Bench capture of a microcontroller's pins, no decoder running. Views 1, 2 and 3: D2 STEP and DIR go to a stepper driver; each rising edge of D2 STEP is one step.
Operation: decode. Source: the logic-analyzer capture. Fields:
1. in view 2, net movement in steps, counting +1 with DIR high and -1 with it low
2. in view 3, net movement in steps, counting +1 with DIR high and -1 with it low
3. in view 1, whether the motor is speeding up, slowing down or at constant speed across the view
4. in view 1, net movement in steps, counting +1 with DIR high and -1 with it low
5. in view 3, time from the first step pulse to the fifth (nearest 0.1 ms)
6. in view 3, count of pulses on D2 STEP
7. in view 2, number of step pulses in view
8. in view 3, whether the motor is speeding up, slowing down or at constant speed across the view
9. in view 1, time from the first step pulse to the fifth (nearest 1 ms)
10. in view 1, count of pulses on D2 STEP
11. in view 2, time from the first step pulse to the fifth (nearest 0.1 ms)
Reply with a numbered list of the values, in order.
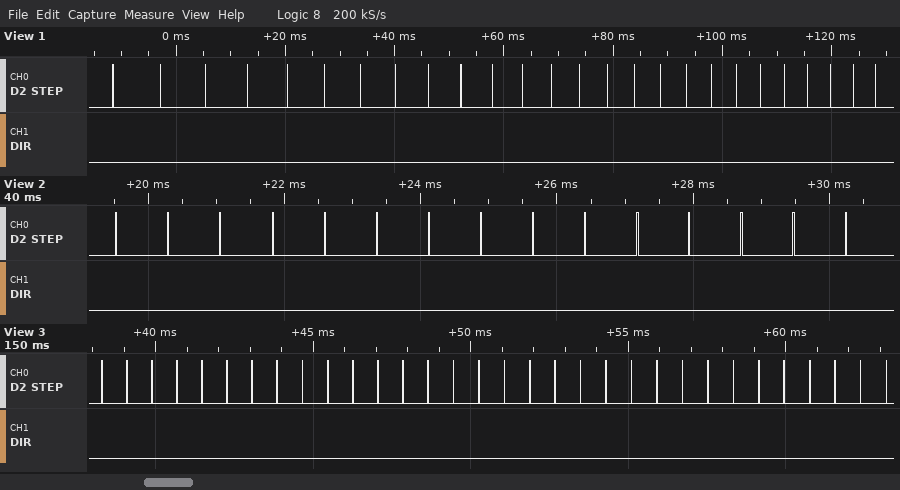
1. -15
2. -32
3. speeding up
4. -26
5. 3.2 ms
6. 32
7. 15
8. constant speed
9. 32 ms
10. 26
11. 3.1 ms
